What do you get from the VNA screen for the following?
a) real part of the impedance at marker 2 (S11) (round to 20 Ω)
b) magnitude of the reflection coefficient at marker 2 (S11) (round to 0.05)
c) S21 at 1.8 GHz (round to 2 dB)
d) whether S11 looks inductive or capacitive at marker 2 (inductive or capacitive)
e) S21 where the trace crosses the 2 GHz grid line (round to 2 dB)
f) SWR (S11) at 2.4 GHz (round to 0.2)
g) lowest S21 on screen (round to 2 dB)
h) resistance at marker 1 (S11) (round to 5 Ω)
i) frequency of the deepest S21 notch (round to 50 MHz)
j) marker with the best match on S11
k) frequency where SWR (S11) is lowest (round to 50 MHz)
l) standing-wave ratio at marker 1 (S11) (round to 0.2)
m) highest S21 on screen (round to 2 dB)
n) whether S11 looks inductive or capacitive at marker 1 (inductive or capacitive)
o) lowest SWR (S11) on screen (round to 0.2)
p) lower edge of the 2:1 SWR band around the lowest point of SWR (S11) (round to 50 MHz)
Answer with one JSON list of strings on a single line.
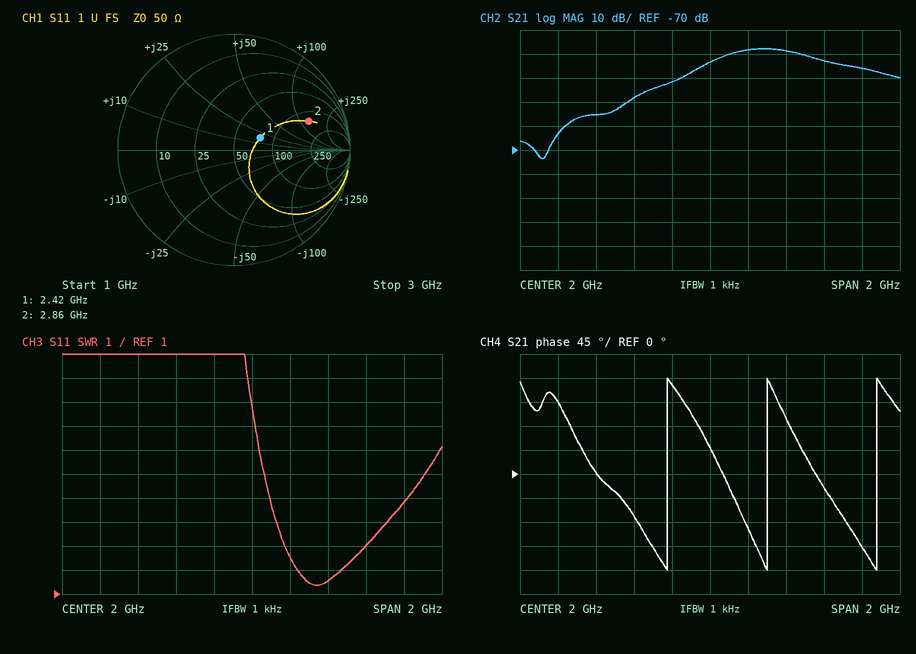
["140 Ω", "0.70", "-42 dB", "inductive", "-34 dB", "1.6", "-74 dB", "75 Ω", "1.10 GHz", "marker 1", "2.35 GHz", "1.6", "-28 dB", "inductive", "1.4", "2.25 GHz"]
